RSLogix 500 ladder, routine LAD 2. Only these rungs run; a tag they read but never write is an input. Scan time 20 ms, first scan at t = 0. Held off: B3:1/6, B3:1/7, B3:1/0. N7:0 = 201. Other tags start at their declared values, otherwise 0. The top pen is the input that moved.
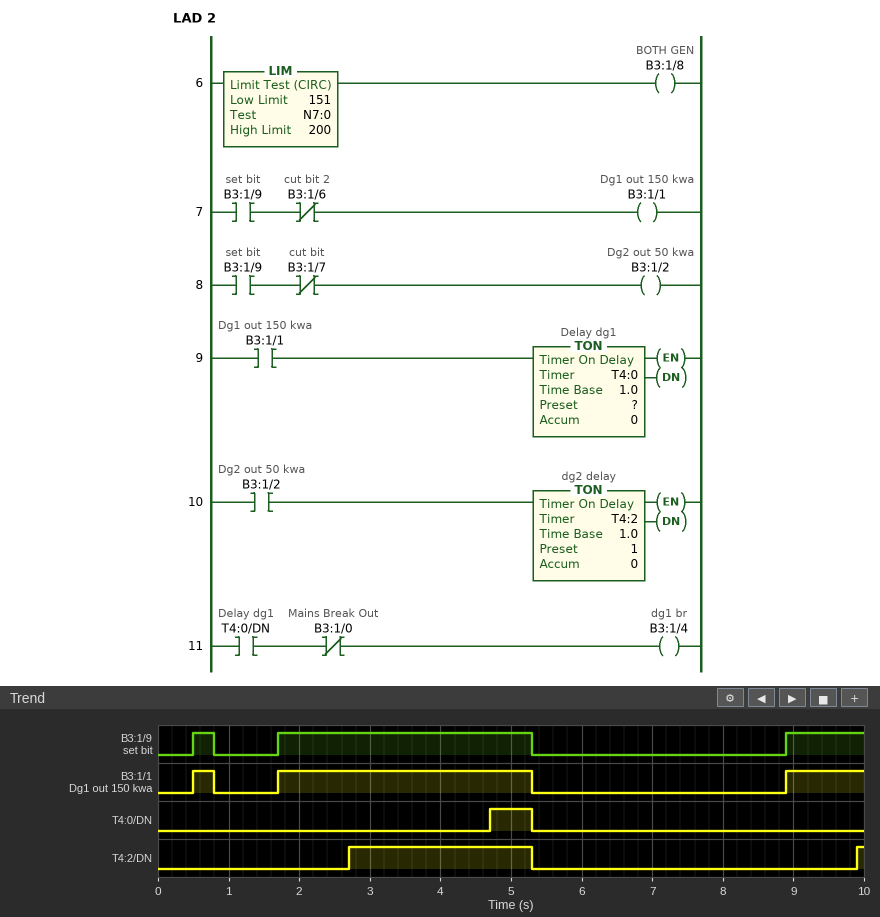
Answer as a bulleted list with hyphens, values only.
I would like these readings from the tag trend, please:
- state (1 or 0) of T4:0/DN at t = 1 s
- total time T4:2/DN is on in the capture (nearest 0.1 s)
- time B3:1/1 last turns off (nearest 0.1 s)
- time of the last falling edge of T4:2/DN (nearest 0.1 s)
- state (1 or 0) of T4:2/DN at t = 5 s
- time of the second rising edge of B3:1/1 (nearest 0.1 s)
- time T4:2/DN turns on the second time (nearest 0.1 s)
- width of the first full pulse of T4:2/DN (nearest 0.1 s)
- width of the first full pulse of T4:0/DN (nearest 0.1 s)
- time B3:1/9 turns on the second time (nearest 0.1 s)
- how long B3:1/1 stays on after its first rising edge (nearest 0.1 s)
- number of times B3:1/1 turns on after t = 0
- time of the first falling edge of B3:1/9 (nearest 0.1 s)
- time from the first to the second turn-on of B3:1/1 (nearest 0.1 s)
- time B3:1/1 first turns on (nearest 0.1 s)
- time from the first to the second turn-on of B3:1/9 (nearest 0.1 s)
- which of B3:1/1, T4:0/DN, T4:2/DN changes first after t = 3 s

- 0
- 2.7 s
- 5.3 s
- 5.3 s
- 1
- 1.7 s
- 9.9 s
- 2.6 s
- 0.6 s
- 1.7 s
- 0.3 s
- 3
- 0.8 s
- 1.2 s
- 0.5 s
- 1.2 s
- T4:0/DN
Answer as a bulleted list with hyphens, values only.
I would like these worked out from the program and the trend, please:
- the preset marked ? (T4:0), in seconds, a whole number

- 3 s
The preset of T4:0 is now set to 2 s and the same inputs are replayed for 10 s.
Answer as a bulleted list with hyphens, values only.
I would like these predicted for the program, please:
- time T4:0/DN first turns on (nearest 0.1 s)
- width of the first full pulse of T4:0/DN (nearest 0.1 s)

- 3.7 s
- 1.6 s
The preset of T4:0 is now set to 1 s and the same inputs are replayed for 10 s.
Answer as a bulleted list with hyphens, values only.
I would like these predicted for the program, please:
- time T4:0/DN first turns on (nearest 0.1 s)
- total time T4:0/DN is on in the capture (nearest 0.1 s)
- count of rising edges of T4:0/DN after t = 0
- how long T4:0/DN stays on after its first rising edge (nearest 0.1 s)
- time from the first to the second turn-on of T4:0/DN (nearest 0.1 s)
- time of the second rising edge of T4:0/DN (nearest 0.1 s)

- 2.7 s
- 2.7 s
- 2
- 2.6 s
- 7.2 s
- 9.9 s
